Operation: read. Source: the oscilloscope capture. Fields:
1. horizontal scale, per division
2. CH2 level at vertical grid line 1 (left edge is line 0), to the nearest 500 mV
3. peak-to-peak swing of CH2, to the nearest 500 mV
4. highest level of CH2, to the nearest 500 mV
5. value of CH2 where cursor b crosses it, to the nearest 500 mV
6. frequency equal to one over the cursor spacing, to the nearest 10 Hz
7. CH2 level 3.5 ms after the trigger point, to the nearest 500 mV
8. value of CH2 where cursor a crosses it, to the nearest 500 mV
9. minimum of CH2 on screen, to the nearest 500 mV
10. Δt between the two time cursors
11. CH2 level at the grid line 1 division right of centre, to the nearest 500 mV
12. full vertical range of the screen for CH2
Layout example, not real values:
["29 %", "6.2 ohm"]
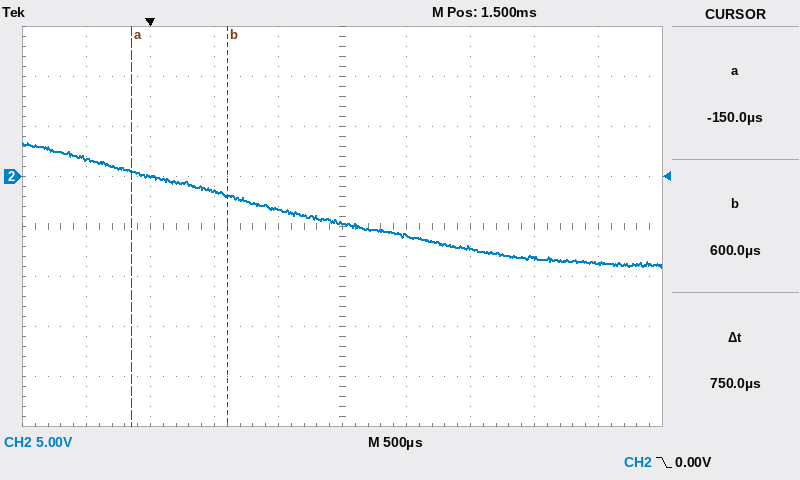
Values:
["500 µs", "2.0 V", "12.5 V", "3.5 V", "-2.0 V", "1.33 kHz", "-8.5 V", "500 mV", "-9.0 V", "750 µs", "-6.0 V", "40 V"]
